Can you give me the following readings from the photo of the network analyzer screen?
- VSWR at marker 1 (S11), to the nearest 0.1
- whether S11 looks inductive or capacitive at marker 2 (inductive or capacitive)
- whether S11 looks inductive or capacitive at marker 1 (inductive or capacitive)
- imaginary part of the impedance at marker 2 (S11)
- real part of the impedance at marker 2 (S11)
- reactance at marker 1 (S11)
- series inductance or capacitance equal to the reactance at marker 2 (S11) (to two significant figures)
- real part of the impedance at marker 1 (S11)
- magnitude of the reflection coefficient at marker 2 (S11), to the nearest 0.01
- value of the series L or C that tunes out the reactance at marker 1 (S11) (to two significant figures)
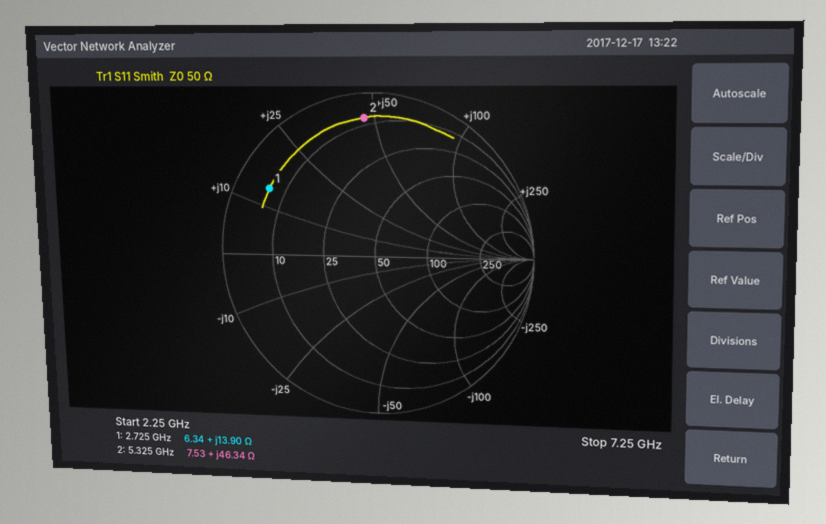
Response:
8.5
inductive
inductive
+46.34 Ω
7.53 Ω
+13.90 Ω
1.4 nH
6.34 Ω
0.85
4.2 pF
